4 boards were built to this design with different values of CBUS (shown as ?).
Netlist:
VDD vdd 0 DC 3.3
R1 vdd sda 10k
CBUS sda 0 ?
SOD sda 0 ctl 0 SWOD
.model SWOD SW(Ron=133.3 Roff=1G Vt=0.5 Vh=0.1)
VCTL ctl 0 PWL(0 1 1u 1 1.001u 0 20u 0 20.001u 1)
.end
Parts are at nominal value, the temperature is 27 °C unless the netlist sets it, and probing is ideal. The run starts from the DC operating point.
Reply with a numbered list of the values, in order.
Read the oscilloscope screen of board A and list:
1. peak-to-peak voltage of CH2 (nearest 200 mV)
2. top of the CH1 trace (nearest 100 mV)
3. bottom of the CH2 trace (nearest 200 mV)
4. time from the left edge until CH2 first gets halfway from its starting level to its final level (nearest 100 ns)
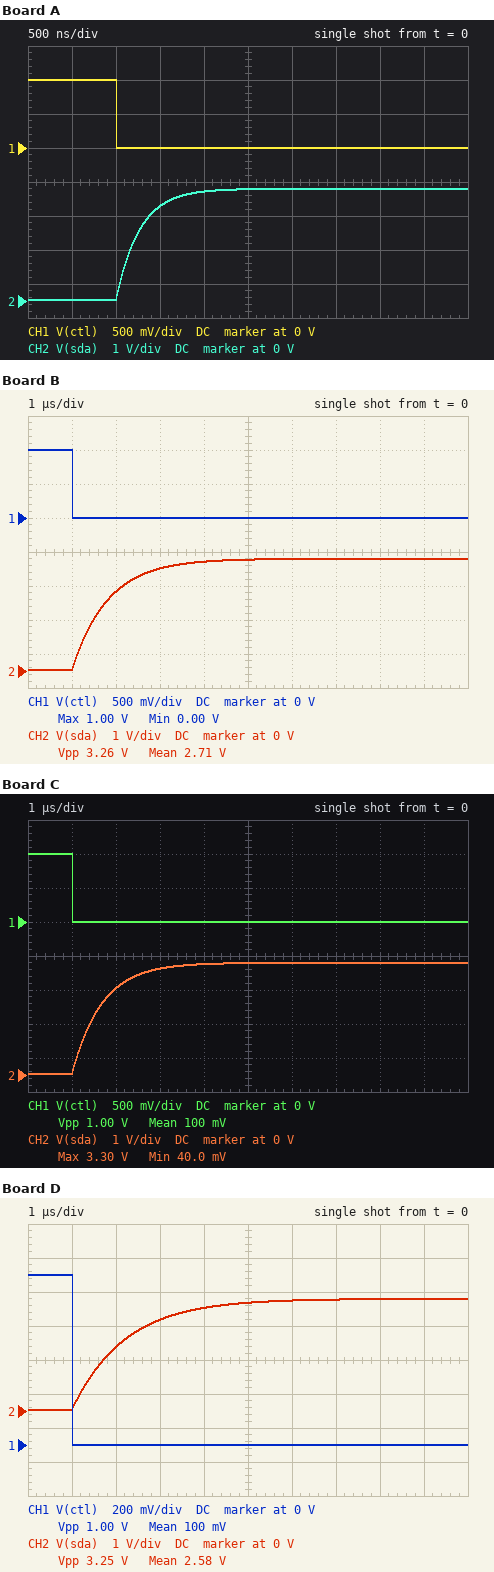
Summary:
1. 3.2 V
2. 1.0 V
3. 0 V
4. 1.2 µs
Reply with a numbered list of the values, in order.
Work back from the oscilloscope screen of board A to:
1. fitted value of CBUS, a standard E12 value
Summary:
1. 27 pF
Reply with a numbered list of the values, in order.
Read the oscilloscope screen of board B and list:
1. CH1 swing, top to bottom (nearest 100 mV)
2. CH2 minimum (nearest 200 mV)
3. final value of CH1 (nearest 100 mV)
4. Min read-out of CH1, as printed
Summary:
1. 1.0 V
2. 0 V
3. 0 V
4. 0.00 V
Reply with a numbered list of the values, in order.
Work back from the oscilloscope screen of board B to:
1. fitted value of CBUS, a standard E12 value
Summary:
1. 82 pF
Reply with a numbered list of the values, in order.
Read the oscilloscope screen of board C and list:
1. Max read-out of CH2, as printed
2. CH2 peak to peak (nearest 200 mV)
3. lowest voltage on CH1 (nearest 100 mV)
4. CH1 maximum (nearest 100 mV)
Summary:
1. 3.30 V
2. 3.2 V
3. 0 V
4. 1.0 V
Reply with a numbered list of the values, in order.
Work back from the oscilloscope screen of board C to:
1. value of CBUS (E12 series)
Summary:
1. 68 pF
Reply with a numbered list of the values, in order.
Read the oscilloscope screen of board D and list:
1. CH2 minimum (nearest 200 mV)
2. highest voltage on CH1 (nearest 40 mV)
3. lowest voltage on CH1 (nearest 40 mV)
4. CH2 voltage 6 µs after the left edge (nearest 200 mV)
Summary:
1. 0 V
2. 1.00 V
3. 0 V
4. 3.2 V
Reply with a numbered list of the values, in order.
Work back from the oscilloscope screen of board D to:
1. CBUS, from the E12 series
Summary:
1. 120 pF
